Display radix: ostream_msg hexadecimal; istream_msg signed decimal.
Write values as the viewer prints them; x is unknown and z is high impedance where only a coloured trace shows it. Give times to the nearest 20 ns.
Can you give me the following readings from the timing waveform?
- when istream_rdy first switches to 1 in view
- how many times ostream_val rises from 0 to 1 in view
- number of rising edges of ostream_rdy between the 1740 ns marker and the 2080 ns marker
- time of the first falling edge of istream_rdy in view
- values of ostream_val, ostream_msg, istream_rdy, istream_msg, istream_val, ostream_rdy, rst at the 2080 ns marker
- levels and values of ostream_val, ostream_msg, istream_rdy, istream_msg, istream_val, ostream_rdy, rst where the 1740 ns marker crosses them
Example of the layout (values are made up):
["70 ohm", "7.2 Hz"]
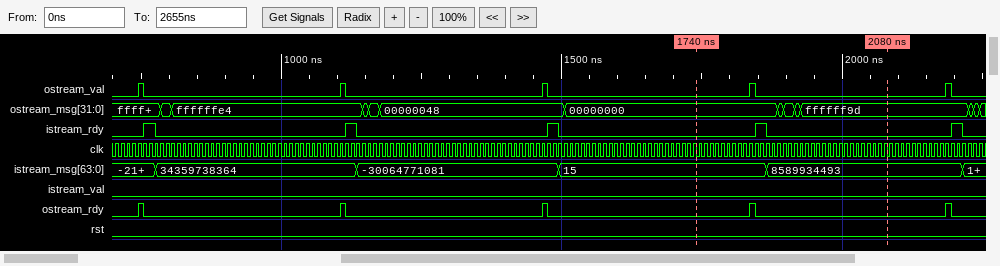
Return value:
["760 ns", "5", "1", "780 ns", "ostream_val=0, ostream_msg=ffffff9d, istream_rdy=0, istream_msg=8589934493, istream_val=0, ostream_rdy=0, rst=0", "ostream_val=0, ostream_msg=00000000, istream_rdy=0, istream_msg=15, istream_val=0, ostream_rdy=0, rst=0"]
